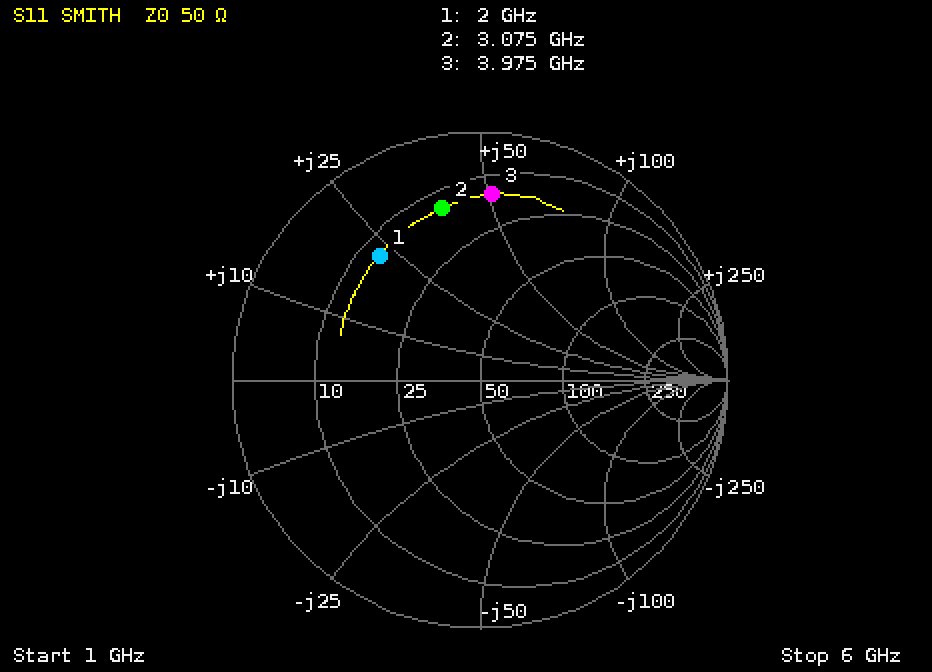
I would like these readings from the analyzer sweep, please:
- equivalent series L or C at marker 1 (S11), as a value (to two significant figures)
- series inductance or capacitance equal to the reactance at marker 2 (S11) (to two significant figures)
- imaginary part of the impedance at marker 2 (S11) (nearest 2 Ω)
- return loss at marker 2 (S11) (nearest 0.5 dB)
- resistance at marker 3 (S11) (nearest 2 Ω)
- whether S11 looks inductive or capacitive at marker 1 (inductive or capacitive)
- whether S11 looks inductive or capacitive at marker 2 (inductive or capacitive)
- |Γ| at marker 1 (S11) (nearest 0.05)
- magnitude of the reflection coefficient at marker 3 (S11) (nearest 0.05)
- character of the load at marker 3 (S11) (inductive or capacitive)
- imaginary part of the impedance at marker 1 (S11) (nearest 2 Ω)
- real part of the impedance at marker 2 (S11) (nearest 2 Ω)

1.8 nH
2.0 nH
+38 Ω
3.0 dB
14 Ω
inductive
inductive
0.65
0.75
inductive
+22 Ω
14 Ω
